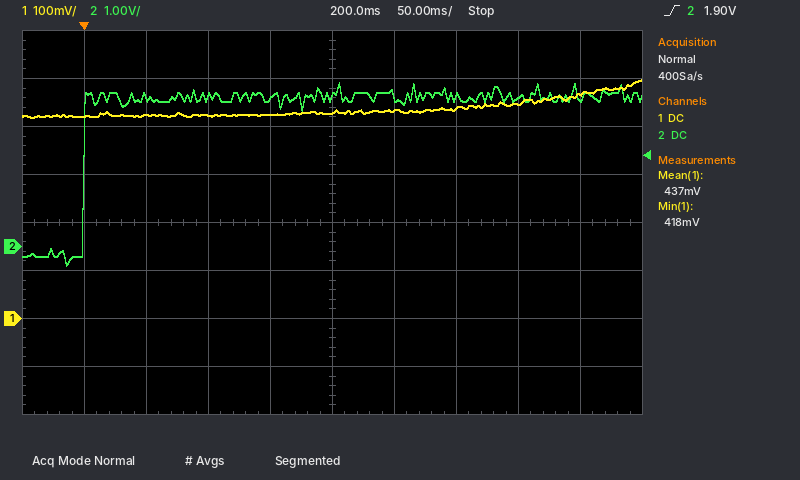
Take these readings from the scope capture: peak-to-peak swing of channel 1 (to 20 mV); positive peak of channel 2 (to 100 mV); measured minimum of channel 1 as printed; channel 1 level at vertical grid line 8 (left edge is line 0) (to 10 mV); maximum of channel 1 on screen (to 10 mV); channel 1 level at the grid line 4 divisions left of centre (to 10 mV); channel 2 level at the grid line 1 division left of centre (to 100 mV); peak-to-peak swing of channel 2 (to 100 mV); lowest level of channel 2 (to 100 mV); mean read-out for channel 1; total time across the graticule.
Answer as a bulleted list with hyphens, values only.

- 80 mV
- 3.4 V
- 418 mV
- 450 mV
- 500 mV
- 420 mV
- 3.1 V
- 3.8 V
- -400 mV
- 437 mV
- 500 ms
